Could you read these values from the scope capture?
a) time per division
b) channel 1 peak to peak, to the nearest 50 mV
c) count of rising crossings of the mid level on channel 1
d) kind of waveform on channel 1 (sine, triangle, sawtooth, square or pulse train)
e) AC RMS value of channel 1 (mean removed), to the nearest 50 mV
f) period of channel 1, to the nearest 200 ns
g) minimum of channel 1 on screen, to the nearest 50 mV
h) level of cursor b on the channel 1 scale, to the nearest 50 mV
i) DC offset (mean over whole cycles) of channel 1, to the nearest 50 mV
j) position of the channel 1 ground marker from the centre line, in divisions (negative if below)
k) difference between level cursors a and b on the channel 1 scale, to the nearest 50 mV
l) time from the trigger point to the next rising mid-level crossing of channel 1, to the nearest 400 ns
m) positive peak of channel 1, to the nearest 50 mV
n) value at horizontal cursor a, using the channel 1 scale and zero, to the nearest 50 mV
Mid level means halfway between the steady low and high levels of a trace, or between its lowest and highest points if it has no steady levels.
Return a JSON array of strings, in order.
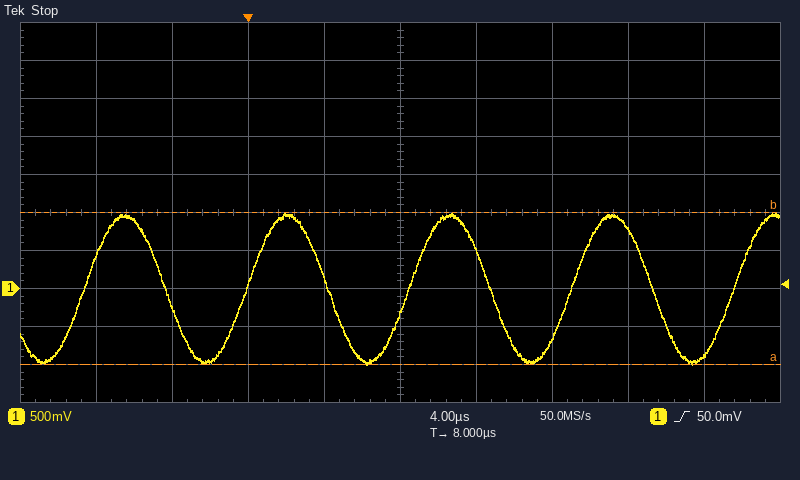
["4 µs", "2.00 V", "5", "sine", "700 mV", "8.6 µs", "-1.00 V", "1.00 V", "0 mV", "-2.0 div", "2.00 V", "8.4 µs", "1.00 V", "-1.00 V"]
